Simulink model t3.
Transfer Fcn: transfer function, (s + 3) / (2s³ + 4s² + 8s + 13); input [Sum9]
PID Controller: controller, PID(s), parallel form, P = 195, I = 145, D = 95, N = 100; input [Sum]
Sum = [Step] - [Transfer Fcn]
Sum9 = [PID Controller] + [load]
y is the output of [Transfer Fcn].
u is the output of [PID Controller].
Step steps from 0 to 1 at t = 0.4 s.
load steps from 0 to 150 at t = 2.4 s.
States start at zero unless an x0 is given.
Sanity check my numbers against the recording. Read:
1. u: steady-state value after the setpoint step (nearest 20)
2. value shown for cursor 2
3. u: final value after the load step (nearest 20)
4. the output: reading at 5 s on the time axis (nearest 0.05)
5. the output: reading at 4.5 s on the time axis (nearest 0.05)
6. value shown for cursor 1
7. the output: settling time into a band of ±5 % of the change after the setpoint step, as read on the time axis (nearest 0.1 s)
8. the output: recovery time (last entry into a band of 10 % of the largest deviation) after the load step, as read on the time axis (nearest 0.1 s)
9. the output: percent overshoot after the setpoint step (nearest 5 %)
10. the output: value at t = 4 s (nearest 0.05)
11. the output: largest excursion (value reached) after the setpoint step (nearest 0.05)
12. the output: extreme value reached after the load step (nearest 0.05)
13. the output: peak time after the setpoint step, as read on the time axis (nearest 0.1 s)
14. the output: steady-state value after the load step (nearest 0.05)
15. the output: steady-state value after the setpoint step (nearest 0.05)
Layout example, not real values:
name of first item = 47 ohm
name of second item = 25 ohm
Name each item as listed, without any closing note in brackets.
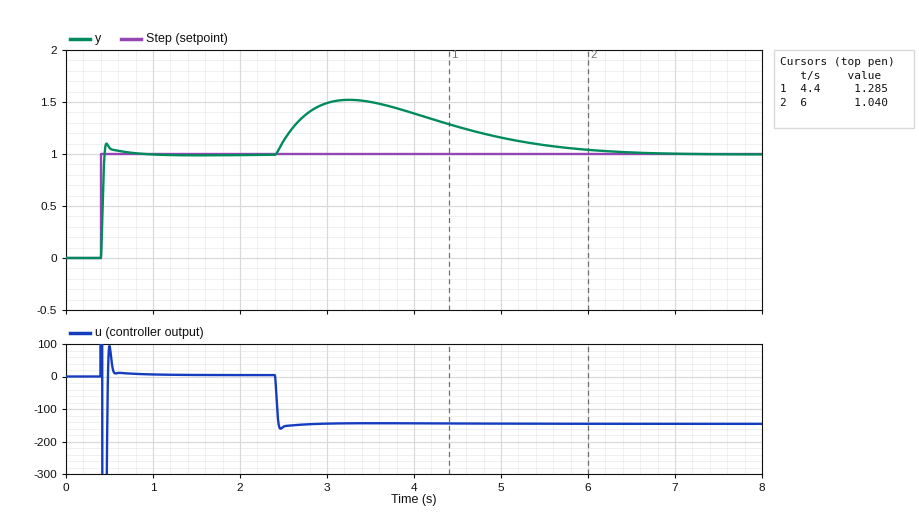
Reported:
u: steady-state value after the setpoint step = 0
value shown for cursor 2 = 1.040
u: final value after the load step = -140
the output: reading at 5 s on the time axis = 1.15
the output: reading at 4.5 s on the time axis = 1.25
value shown for cursor 1 = 1.285
the output: settling time into a band of ±5 % of the change after the setpoint step, as read on the time axis = 0.5 s
the output: recovery time (last entry into a band of 10 % of the largest deviation) after the load step, as read on the time axis = 5.8 s
the output: percent overshoot after the setpoint step = 10 %
the output: value at t = 4 s = 1.40
the output: largest excursion (value reached) after the setpoint step = 1.10
the output: extreme value reached after the load step = 1.50
the output: peak time after the setpoint step, as read on the time axis = 0.5 s
the output: steady-state value after the load step = 1.00
the output: steady-state value after the setpoint step = 1.00
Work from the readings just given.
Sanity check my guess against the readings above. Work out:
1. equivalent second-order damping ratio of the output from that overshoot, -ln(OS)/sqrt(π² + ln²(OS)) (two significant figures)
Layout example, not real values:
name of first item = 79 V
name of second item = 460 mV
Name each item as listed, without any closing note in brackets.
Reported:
equivalent second-order damping ratio of the output from that overshoot, -ln(OS)/sqrt(π² + ln²(OS)) = 0.59
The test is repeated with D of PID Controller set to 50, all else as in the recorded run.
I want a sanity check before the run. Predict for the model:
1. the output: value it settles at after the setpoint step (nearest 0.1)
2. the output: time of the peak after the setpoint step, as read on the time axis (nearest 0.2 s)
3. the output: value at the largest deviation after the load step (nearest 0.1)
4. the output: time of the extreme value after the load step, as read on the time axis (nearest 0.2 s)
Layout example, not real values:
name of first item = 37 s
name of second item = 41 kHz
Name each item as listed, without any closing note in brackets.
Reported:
the output: value it settles at after the setpoint step = 1.0
the output: time of the peak after the setpoint step, as read on the time axis = 0.6 s
the output: value at the largest deviation after the load step = 1.6
the output: time of the extreme value after the load step, as read on the time axis = 3.0 s
